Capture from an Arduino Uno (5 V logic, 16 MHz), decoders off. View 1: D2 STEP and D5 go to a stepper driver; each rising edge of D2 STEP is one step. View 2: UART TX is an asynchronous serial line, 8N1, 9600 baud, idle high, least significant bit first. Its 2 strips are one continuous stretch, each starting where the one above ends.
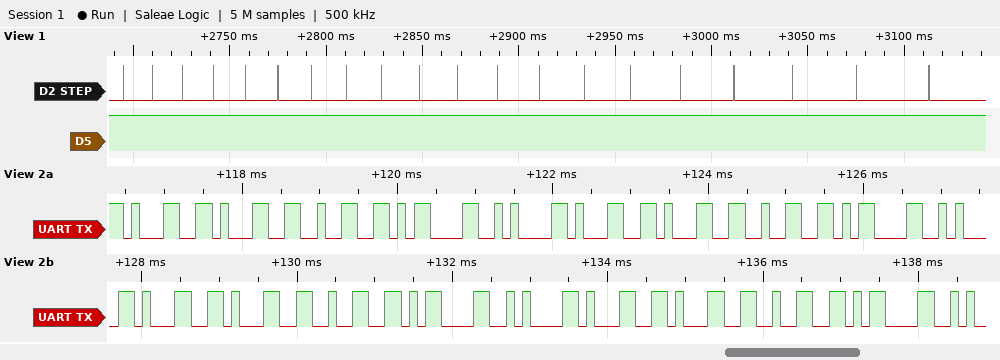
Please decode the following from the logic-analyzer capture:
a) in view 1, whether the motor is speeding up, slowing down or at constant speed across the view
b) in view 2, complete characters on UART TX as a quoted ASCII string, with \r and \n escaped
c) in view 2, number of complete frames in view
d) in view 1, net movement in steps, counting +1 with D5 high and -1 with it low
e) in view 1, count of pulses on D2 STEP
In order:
slowing down
"112\r\n112\r\n112\r\n112\r"
19
+20
20
